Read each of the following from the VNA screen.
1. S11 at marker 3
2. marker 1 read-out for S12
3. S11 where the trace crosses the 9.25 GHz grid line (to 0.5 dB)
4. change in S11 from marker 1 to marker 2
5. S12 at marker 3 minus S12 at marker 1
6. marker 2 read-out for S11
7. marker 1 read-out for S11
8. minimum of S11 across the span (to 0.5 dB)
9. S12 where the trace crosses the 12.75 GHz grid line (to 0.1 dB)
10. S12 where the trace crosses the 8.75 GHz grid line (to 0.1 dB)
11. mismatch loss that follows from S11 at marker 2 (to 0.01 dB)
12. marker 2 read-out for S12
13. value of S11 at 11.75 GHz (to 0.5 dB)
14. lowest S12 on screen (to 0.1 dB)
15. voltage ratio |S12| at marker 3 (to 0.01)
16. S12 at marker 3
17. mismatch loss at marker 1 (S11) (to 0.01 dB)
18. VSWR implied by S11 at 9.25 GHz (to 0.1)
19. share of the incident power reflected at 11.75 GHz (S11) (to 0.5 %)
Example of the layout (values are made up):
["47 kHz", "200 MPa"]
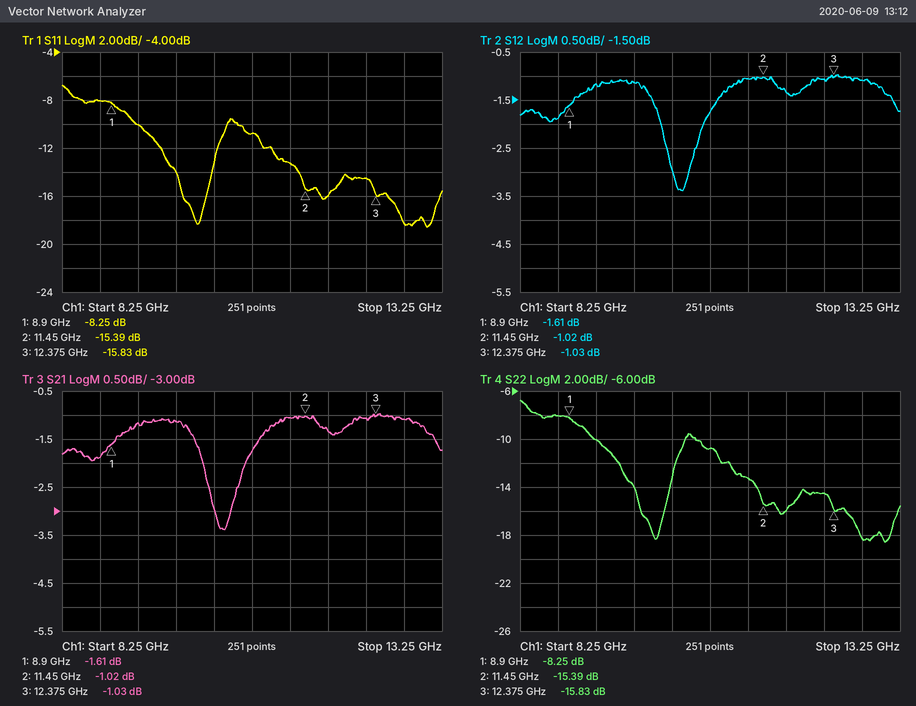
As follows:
["-15.83 dB", "-1.61 dB", "-10.0 dB", "-7.14 dB", "0.58 dB", "-15.39 dB", "-8.25 dB", "-18.5 dB", "-1.1 dB", "-1.9 dB", "0.13 dB", "-1.02 dB", "-16.0 dB", "-3.4 dB", "0.89", "-1.03 dB", "0.70 dB", "1.9", "2.5 %"]
